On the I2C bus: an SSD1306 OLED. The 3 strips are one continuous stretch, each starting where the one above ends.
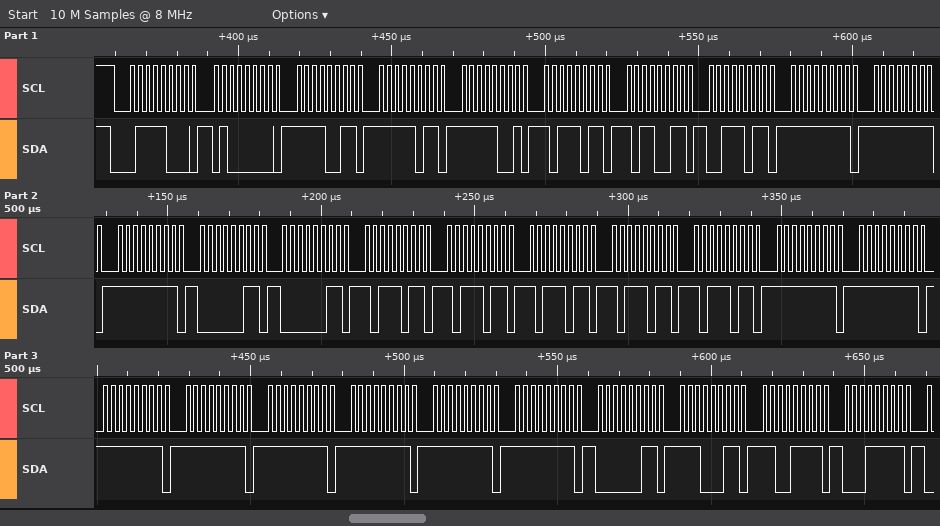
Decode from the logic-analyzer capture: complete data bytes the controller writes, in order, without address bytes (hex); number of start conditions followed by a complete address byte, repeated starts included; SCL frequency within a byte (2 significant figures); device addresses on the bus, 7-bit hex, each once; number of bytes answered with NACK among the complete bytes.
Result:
40 F3 FB F9 BB B3 3B FF FF FF 03 03 BB BB BB BB BB FF FF FF FF FF FF FF FF 03 E3 CF 1F
1
400 kHz
0x3C
0
